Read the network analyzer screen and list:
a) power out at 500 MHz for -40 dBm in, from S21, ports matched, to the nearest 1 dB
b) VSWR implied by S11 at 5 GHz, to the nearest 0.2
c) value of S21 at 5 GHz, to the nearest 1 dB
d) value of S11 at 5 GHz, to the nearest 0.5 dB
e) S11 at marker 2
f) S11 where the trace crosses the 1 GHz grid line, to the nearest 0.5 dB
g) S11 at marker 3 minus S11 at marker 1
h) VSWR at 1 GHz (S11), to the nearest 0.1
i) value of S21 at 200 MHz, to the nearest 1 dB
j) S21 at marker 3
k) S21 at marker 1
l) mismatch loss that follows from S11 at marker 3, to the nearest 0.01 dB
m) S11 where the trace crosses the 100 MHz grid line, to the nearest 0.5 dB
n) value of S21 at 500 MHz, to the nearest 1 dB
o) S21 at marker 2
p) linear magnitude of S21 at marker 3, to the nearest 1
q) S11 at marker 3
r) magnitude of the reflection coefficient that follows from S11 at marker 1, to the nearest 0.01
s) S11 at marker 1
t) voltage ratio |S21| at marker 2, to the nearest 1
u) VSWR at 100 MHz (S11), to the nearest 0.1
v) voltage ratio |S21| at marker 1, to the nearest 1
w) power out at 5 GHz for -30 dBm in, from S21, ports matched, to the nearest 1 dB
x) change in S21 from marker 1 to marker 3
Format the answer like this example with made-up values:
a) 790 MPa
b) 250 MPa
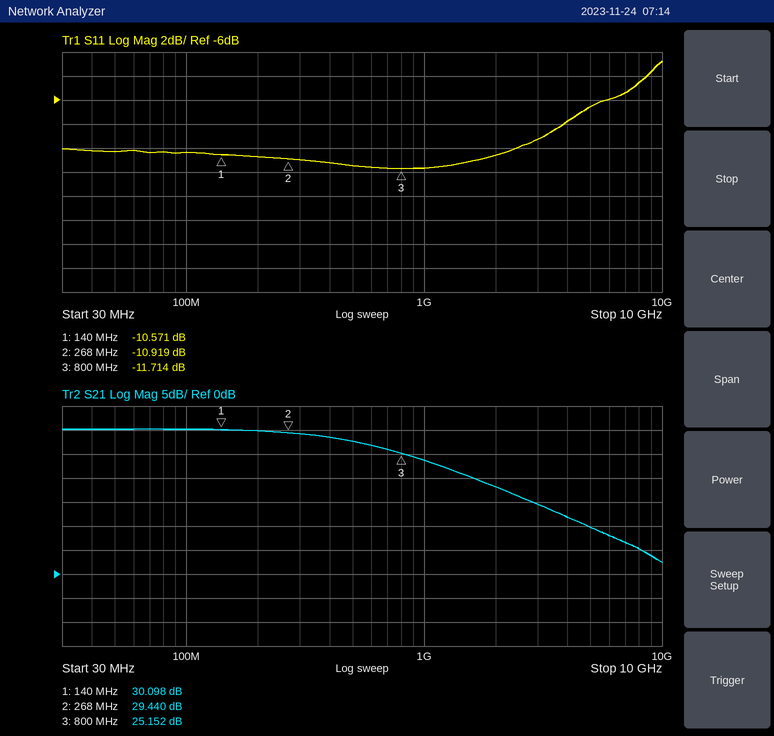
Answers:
a) -12 dBm
b) 2.8
c) 10 dB
d) -6.5 dB
e) -10.919 dB
f) -11.5 dB
g) -1.143 dB
h) 1.7
i) 30 dB
j) 25.152 dB
k) 30.098 dB
l) 0.30 dB
m) -10.5 dB
n) 28 dB
o) 29.440 dB
p) 18
q) -11.714 dB
r) 0.30
s) -10.571 dB
t) 30
u) 1.9
v) 32
w) -20 dBm
x) -4.946 dB
